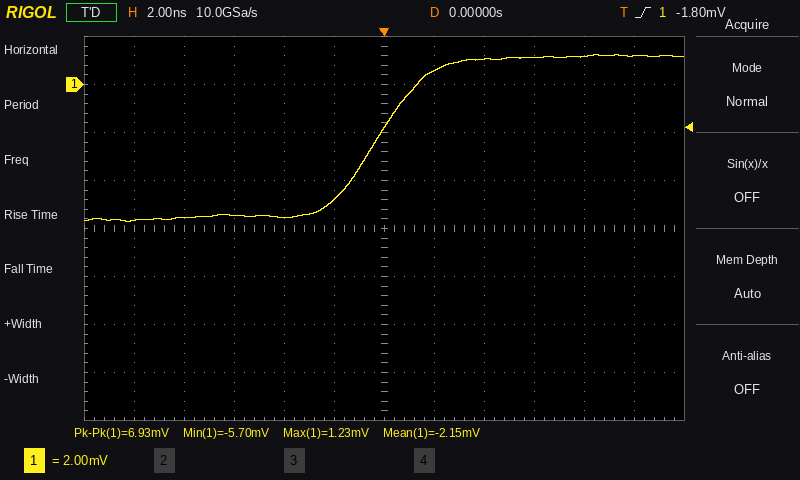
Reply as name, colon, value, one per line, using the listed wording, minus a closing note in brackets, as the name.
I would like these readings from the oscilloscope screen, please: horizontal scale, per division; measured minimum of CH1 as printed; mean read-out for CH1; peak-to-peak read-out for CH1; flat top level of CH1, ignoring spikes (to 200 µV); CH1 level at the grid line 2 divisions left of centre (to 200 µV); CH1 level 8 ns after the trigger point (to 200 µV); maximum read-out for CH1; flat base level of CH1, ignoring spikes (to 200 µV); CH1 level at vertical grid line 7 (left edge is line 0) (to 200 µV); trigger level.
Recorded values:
horizontal scale, per division: 2 ns
measured minimum of CH1 as printed: -5.70 mV
mean read-out for CH1: -2.15 mV
peak-to-peak read-out for CH1: 6.93 mV
flat top level of CH1, ignoring spikes: 1.2 mV
CH1 level at the grid line 2 divisions left of centre: -5.6 mV
CH1 level 8 ns after the trigger point: 1.2 mV
maximum read-out for CH1: 1.23 mV
flat base level of CH1, ignoring spikes: -5.6 mV
CH1 level at vertical grid line 7 (left edge is line 0): 600 µV
trigger level: -1.80 mV
